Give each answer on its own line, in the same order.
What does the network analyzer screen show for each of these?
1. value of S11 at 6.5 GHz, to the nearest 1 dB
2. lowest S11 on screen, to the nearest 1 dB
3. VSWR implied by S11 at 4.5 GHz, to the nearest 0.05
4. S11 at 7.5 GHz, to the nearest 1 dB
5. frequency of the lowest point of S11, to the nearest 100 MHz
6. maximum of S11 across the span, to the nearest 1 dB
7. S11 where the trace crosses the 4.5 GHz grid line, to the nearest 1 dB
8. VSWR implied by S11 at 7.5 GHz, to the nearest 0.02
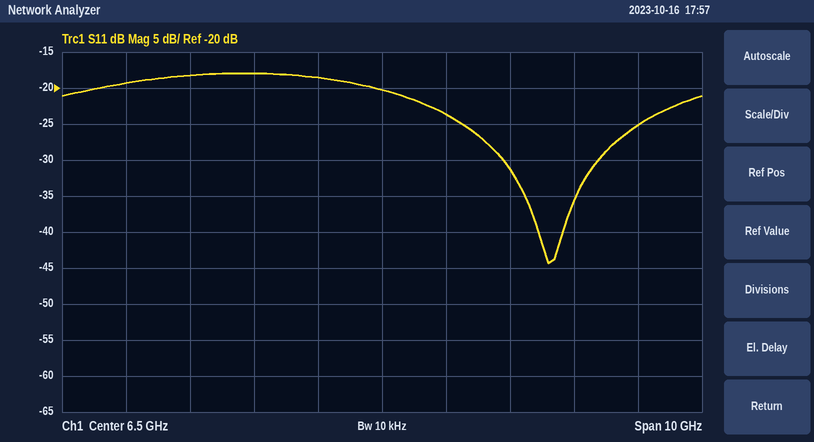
-20 dB
-44 dB
1.30
-24 dB
9.1 GHz
-18 dB
-18 dB
1.14
